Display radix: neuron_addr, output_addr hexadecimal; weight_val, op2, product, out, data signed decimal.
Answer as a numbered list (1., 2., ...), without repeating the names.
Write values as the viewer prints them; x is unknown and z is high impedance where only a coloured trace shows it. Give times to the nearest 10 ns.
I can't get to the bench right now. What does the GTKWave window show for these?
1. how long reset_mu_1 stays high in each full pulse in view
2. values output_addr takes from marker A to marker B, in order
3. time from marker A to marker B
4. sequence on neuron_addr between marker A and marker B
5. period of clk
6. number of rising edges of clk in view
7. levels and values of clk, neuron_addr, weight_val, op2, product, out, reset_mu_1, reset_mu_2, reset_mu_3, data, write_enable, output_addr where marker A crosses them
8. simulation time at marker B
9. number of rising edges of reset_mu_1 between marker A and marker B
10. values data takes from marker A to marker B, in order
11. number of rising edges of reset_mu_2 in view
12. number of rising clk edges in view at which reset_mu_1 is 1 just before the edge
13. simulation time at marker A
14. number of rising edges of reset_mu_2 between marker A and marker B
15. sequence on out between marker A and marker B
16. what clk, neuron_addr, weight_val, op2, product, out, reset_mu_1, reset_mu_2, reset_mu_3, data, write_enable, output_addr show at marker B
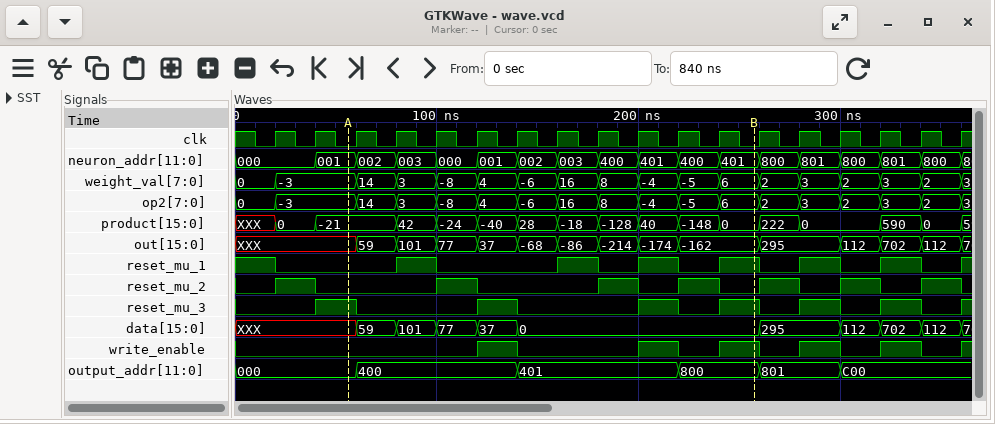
1. 20 ns, 20 ns, 20 ns, 20 ns, 20 ns, 20 ns
2. 000, 400, 401, 800
3. 200 ns
4. 001, 002, 003, 000, 001, 002, 003, 400, 401, 400, 401
5. 20 ns
6. 18
7. clk=0, neuron_addr=001, weight_val=-3, op2=-3, product=-21, out=XXX, reset_mu_1=0, reset_mu_2=0, reset_mu_3=1, data=XXX, write_enable=0, output_addr=000
8. 260 ns
9. 4
10. XXX, 59, 101, 77, 37, 0
11. 7
12. 7
13. 60 ns
14. 3
15. XXX, 59, 101, 77, 37, -68, -86, -214, -174, -162
16. clk=0, neuron_addr=401, weight_val=6, op2=6, product=0, out=-162, reset_mu_1=1, reset_mu_2=0, reset_mu_3=1, data=0, write_enable=1, output_addr=800
